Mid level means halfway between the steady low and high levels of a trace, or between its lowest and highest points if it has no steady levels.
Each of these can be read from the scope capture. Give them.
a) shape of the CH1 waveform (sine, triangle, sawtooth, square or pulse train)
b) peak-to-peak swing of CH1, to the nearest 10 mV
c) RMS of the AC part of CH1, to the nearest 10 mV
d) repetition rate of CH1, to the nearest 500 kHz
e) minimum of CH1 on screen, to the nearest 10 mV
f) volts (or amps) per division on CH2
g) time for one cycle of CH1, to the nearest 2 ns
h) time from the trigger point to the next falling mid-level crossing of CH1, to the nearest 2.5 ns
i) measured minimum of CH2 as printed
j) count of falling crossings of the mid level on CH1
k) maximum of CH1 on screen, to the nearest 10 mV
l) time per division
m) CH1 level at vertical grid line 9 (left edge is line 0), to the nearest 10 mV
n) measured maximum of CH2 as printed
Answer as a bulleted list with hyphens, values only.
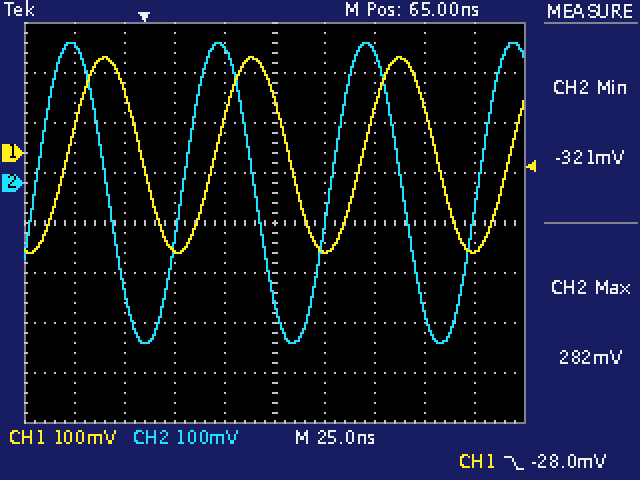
- sine
- 390 mV
- 140 mV
- 13.5 MHz
- -200 mV
- 100 mV
- 74 ns
- 72.5 ns
- -321 mV
- 3
- 190 mV
- 25 ns
- -200 mV
- 282 mV
